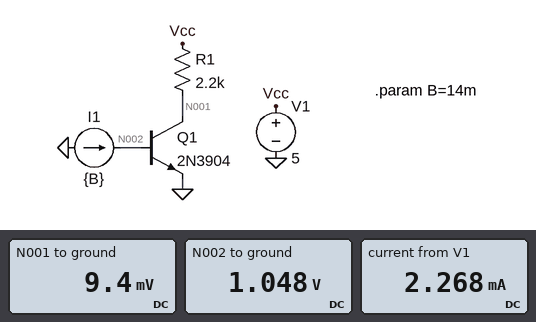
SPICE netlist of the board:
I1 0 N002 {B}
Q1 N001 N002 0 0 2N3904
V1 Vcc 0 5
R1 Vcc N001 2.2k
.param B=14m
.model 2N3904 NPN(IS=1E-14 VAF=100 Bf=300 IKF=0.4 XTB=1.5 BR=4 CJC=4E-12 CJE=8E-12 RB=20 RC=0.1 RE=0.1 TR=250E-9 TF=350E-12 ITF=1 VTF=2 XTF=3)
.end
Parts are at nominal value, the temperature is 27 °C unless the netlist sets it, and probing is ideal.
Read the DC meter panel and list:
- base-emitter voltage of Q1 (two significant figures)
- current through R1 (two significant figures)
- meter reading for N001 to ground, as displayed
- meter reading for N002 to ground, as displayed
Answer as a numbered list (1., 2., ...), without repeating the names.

1. 1.0 V
2. 2.3 mA
3. 9.4 mV
4. 1.048 V
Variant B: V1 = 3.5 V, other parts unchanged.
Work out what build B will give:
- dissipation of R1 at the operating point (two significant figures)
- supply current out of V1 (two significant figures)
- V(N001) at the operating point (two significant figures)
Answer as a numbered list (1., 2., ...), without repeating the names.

1. 5.5 mW
2. 1.6 mA
3. 9.0 mV
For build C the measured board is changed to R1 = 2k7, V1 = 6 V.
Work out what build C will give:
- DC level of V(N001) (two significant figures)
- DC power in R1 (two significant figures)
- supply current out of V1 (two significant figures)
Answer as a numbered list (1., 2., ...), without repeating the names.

1. 9.4 mV
2. 13 mW
3. 2.2 mA
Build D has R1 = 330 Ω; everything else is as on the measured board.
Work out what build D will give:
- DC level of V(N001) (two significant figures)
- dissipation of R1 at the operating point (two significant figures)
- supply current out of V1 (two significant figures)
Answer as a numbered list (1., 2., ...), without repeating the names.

1. 17 mV
2. 75 mW
3. 15 mA
